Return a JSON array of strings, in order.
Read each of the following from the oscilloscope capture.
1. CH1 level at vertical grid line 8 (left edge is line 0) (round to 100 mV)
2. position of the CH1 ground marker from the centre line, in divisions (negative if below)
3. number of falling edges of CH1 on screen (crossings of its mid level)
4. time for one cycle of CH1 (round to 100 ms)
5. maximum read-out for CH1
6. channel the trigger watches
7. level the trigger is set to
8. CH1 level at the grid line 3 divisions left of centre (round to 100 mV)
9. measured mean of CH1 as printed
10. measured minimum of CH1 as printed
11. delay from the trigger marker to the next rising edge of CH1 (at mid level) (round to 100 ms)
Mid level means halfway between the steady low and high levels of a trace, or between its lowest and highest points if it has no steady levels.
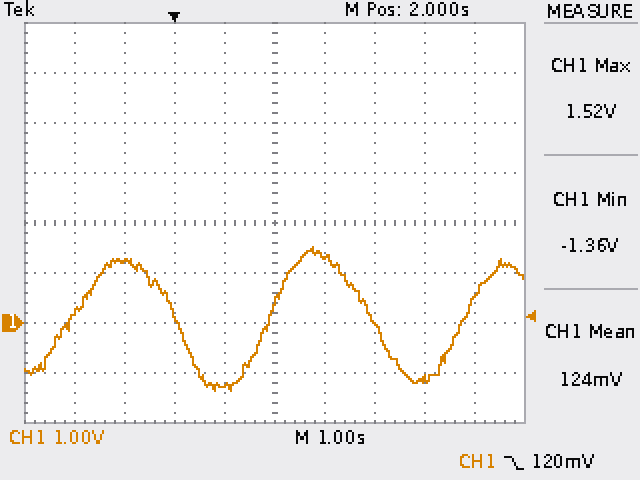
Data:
["-1.1 V", "-2.0 div", "2", "3.9 s", "1.52 V", "CH1", "120 mV", "1.2 V", "124 mV", "-1.36 V", "1.9 s"]
